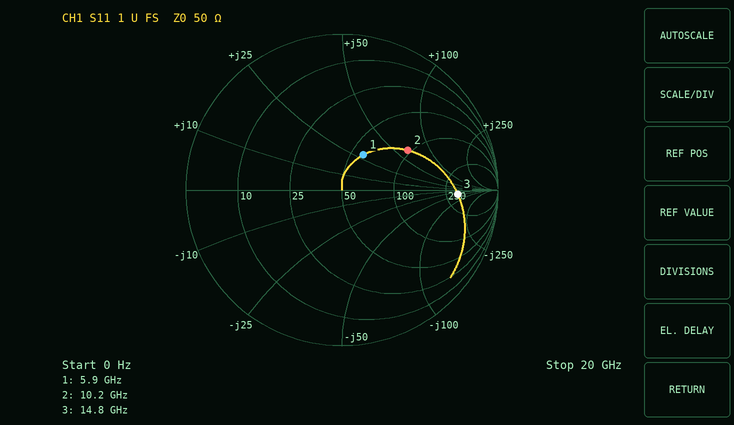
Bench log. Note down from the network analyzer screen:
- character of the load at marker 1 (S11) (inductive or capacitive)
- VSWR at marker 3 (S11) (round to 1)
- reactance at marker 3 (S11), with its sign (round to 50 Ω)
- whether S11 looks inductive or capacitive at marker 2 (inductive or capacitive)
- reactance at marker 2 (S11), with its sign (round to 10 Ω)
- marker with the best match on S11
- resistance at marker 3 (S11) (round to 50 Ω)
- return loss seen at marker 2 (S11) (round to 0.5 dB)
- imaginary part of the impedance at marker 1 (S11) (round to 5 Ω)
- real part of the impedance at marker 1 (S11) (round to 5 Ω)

inductive
7
-50 Ω
inductive
+60 Ω
marker 1
350 Ω
6.0 dB
+30 Ω
60 Ω
